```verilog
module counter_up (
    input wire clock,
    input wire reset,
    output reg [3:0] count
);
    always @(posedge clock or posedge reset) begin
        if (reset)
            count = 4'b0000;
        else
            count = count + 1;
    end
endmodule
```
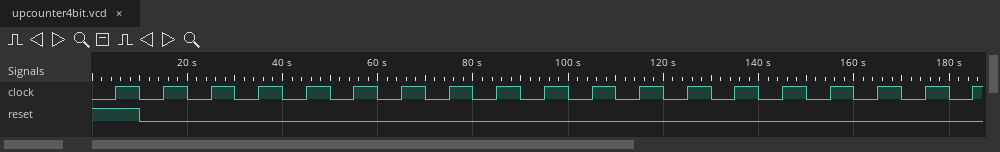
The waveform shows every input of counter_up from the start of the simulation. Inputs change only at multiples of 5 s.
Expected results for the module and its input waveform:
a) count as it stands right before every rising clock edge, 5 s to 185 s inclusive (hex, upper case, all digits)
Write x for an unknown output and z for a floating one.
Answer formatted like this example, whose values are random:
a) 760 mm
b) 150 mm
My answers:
a) 0, 0, 1, 2, 3, 4, 5, 6, 7, 8, 9, A, B, C, D, E, F, 0, 1
